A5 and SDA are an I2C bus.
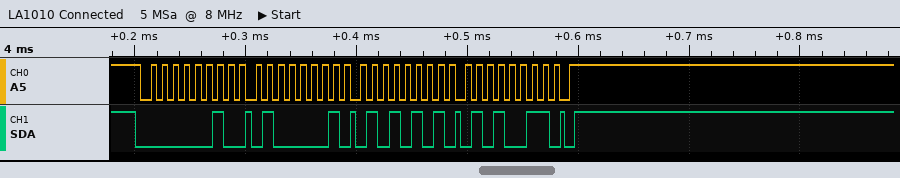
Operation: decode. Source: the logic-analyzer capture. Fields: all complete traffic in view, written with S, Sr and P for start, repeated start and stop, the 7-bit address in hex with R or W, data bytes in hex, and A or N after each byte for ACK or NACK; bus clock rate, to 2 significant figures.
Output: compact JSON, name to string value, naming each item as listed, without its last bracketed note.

{"all complete traffic in view, written with S, Sr and P for start, repeated start and stop, the 7-bit address in hex with R or W, data bytes in hex, and A or N after each byte for ACK or NACK": "S 01W A 41 A 55 A 53 A P", "bus clock rate, to 2 significant figures": "100 kHz"}
